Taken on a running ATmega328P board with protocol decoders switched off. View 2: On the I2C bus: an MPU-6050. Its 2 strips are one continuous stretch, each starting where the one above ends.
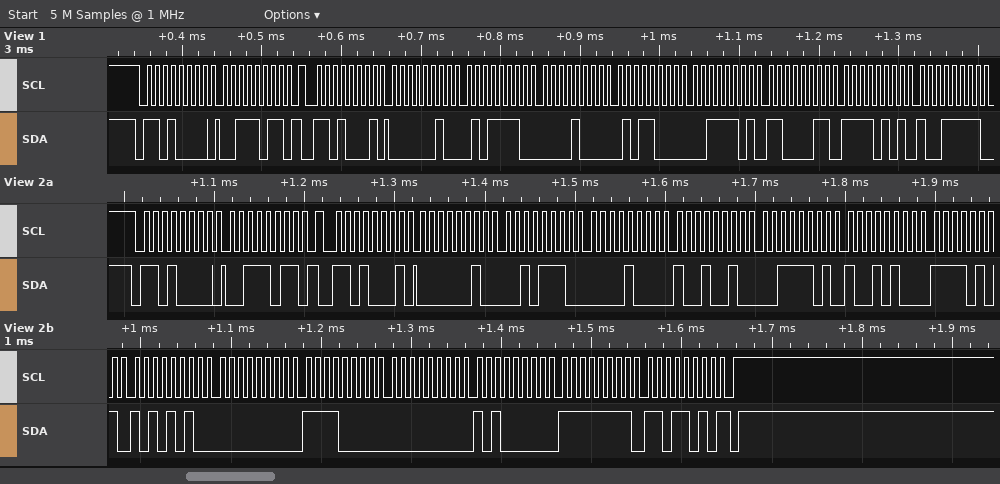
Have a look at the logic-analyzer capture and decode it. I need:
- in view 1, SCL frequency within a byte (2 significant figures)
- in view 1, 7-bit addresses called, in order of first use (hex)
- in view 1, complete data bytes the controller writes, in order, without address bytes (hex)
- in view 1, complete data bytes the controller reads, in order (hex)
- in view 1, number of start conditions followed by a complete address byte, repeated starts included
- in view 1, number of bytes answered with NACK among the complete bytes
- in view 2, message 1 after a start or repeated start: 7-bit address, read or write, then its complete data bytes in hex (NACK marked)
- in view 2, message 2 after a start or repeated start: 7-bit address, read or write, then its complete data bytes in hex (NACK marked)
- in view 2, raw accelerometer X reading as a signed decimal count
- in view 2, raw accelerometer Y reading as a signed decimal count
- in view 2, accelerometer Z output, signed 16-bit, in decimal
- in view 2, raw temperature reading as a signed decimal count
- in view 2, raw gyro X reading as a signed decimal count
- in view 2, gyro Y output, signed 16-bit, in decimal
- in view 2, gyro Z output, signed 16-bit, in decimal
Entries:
100 kHz
0x68
3B
02 5E 08 58 3D C3 F5 9F
2
0
0x68 write: 3B
0x68 read: 02 2E 08 92 3D 94 F5 AA 00 F0 00 A0 FF DA NACK
558
2194
15764
-2646
240
160
-38
